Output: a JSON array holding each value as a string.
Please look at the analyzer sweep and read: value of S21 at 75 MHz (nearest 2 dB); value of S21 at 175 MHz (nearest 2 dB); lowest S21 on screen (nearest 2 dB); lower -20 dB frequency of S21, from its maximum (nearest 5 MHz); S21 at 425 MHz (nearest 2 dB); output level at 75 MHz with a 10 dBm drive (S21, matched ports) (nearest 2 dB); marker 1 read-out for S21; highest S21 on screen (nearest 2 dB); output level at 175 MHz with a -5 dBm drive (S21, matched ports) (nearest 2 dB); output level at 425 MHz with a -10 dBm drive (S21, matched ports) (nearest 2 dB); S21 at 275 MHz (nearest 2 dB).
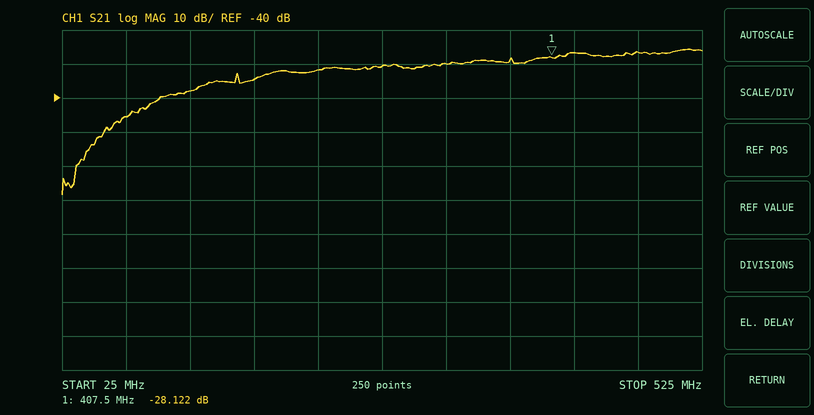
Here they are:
["-46 dB", "-34 dB", "-68 dB", "75 MHz", "-26 dB", "-36 dBm", "-28.122 dB", "-26 dB", "-40 dBm", "-36 dBm", "-30 dB"]
